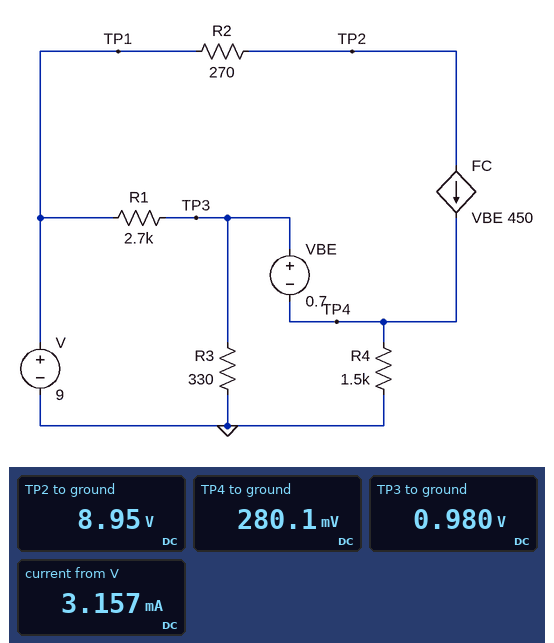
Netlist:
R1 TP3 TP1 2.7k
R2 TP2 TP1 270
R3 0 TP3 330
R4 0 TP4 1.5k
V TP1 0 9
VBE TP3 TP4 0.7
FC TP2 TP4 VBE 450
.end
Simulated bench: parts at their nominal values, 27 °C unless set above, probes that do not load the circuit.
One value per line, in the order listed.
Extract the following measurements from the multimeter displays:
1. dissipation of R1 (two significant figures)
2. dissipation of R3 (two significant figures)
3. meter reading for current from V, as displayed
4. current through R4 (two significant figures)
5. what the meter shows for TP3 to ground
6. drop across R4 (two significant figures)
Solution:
24 mW
2.9 mW
3.157 mA
190 µA
0.980 V
280 mV
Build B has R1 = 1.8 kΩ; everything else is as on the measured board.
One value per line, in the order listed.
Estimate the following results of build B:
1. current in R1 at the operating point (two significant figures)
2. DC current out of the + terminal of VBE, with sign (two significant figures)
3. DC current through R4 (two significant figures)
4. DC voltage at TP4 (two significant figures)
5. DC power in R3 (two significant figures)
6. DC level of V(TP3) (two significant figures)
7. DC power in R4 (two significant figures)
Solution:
4.2 mA
-1.0 µA
460 µA
690 mV
5.9 mW
1.4 V
320 µW
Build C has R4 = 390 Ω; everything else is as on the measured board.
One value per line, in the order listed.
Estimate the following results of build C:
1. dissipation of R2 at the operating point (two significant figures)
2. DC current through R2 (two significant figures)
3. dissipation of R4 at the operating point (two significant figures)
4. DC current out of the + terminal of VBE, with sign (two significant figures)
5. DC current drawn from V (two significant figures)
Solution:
140 µW
720 µA
200 µW
-1.6 µA
3.7 mA
